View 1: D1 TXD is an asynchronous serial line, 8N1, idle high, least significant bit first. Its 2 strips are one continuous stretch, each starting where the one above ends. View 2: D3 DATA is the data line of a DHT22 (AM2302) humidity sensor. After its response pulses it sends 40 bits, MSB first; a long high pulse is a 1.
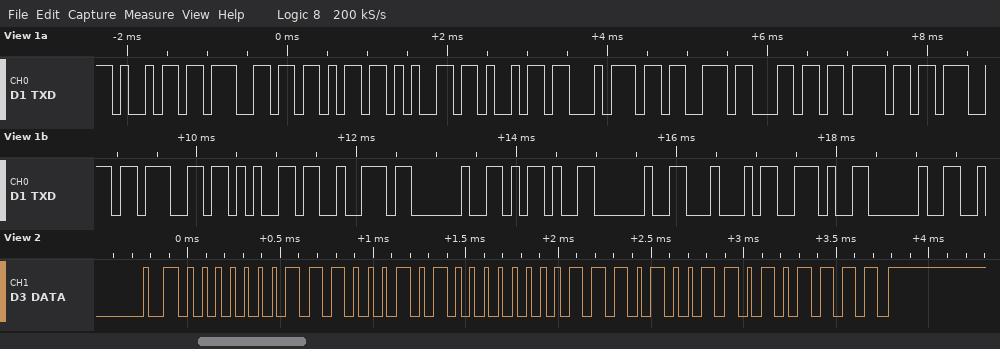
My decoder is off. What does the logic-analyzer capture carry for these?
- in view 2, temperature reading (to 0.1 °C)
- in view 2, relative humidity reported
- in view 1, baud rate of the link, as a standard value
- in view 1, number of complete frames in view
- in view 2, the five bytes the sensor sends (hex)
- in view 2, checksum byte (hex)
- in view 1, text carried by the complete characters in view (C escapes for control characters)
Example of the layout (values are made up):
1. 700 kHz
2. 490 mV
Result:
1. 23.3 °C
2. 45.3 %
3. 9600 baud
4. 19
5. 01 C5 00 E9 AF
6. 0xAF
7. "igkeitslogger - D. "
